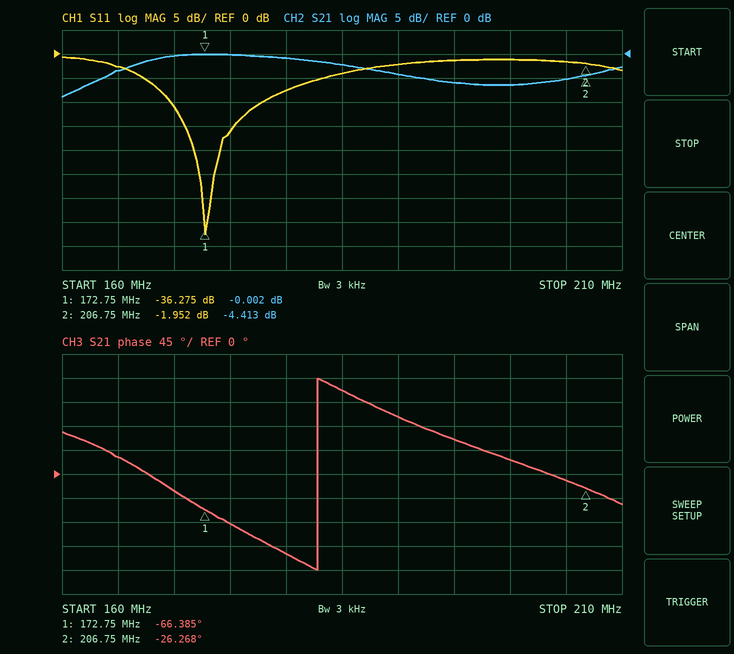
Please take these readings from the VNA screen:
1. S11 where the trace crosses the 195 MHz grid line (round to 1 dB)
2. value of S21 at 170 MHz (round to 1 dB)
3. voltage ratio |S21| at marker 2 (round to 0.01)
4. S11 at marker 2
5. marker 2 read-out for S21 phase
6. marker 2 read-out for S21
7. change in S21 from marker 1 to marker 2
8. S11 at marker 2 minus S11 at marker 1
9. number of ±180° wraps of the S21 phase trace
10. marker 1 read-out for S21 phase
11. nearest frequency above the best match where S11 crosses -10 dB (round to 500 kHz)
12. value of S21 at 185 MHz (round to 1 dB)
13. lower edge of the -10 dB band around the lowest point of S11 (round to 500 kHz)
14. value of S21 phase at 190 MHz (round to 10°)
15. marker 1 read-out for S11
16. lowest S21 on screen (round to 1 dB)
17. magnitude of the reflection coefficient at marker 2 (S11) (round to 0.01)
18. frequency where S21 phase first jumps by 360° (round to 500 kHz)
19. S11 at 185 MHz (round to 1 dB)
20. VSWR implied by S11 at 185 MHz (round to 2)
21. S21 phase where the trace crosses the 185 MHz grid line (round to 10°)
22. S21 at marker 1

-1 dB
0 dB
0.60
-1.952 dB
-26.268°
-4.413 dB
-4.411 dB
34.323 dB
1
-66.385°
178.0 MHz
-2 dB
169.5 MHz
110°
-36.275 dB
-9 dB
0.80
183.0 MHz
-4 dB
4
160°
-0.002 dB
